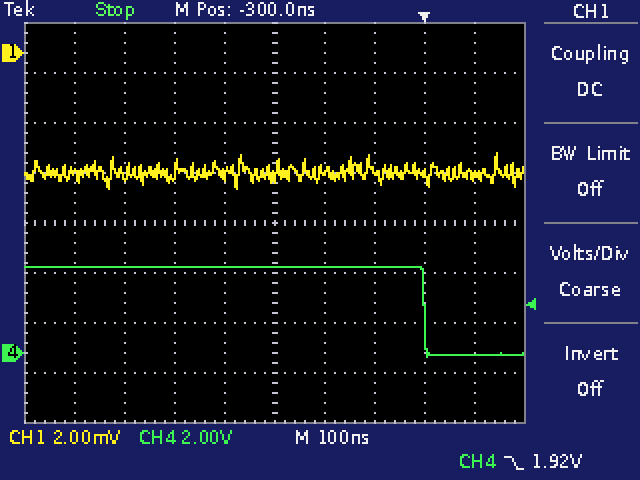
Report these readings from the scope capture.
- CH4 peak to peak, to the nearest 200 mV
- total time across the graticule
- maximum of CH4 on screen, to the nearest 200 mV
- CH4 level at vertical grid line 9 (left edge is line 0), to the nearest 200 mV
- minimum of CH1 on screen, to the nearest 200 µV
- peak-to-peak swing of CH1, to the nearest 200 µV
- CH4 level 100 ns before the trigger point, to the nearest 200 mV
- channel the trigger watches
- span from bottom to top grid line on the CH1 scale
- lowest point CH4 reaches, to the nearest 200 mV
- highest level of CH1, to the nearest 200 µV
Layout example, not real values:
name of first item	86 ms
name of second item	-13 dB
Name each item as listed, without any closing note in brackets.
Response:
CH4 peak to peak, to the nearest 200 mV	3.6 V
total time across the graticule	1 µs
maximum of CH4 on screen, to the nearest 200 mV	3.4 V
CH4 level at vertical grid line 9 (left edge is line 0), to the nearest 200 mV	0.0 V
minimum of CH1 on screen, to the nearest 200 µV	-5.4 mV
peak-to-peak swing of CH1, to the nearest 200 µV	1.4 mV
CH4 level 100 ns before the trigger point, to the nearest 200 mV	3.4 V
channel the trigger watches	CH4
span from bottom to top grid line on the CH1 scale	16 mV
lowest point CH4 reaches, to the nearest 200 mV	-200 mV
highest level of CH1, to the nearest 200 µV	-4.0 mV
